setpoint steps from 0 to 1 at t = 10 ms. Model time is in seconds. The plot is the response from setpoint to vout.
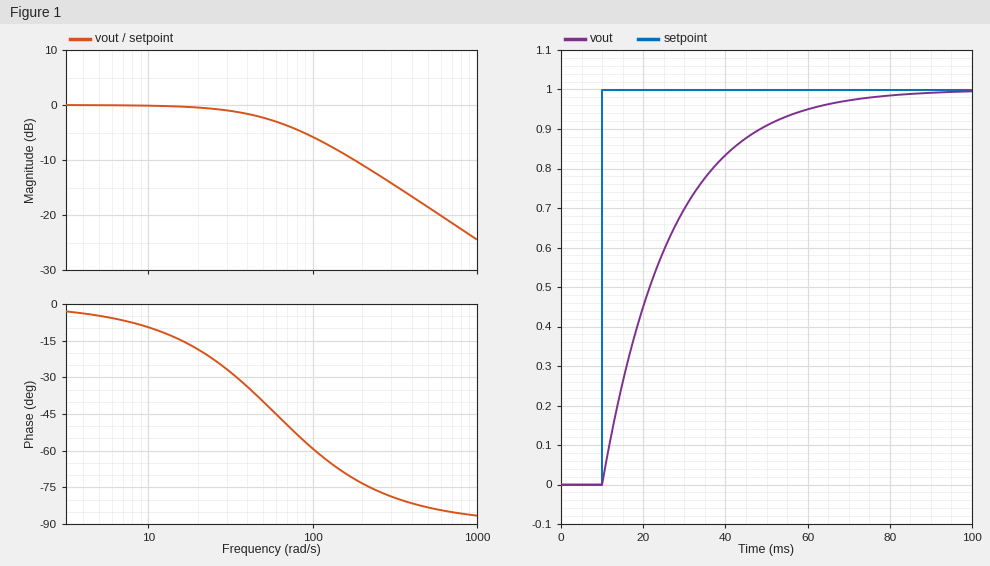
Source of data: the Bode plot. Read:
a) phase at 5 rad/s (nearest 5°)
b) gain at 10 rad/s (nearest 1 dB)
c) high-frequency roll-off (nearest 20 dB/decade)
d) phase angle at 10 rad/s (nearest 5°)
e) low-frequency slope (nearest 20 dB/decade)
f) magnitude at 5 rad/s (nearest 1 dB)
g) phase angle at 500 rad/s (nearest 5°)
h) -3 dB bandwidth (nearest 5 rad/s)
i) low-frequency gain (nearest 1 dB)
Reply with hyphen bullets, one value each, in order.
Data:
- -5°
- 0 dB
- -20 dB/decade
- -10°
- 0 dB/decade
- 0 dB
- -85°
- 60 rad/s
- 0 dB
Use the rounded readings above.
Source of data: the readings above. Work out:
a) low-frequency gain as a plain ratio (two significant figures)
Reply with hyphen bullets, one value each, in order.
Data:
- 1.0
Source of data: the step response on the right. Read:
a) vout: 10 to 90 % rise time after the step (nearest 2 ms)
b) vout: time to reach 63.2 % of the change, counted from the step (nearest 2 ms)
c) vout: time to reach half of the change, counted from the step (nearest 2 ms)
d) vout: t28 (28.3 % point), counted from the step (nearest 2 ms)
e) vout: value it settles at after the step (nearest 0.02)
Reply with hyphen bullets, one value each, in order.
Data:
- 36 ms
- 16 ms
- 12 ms
- 6 ms
- 1.00
